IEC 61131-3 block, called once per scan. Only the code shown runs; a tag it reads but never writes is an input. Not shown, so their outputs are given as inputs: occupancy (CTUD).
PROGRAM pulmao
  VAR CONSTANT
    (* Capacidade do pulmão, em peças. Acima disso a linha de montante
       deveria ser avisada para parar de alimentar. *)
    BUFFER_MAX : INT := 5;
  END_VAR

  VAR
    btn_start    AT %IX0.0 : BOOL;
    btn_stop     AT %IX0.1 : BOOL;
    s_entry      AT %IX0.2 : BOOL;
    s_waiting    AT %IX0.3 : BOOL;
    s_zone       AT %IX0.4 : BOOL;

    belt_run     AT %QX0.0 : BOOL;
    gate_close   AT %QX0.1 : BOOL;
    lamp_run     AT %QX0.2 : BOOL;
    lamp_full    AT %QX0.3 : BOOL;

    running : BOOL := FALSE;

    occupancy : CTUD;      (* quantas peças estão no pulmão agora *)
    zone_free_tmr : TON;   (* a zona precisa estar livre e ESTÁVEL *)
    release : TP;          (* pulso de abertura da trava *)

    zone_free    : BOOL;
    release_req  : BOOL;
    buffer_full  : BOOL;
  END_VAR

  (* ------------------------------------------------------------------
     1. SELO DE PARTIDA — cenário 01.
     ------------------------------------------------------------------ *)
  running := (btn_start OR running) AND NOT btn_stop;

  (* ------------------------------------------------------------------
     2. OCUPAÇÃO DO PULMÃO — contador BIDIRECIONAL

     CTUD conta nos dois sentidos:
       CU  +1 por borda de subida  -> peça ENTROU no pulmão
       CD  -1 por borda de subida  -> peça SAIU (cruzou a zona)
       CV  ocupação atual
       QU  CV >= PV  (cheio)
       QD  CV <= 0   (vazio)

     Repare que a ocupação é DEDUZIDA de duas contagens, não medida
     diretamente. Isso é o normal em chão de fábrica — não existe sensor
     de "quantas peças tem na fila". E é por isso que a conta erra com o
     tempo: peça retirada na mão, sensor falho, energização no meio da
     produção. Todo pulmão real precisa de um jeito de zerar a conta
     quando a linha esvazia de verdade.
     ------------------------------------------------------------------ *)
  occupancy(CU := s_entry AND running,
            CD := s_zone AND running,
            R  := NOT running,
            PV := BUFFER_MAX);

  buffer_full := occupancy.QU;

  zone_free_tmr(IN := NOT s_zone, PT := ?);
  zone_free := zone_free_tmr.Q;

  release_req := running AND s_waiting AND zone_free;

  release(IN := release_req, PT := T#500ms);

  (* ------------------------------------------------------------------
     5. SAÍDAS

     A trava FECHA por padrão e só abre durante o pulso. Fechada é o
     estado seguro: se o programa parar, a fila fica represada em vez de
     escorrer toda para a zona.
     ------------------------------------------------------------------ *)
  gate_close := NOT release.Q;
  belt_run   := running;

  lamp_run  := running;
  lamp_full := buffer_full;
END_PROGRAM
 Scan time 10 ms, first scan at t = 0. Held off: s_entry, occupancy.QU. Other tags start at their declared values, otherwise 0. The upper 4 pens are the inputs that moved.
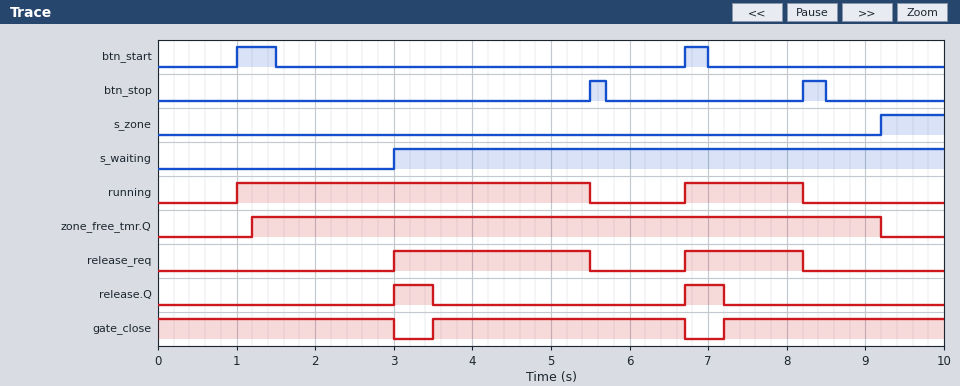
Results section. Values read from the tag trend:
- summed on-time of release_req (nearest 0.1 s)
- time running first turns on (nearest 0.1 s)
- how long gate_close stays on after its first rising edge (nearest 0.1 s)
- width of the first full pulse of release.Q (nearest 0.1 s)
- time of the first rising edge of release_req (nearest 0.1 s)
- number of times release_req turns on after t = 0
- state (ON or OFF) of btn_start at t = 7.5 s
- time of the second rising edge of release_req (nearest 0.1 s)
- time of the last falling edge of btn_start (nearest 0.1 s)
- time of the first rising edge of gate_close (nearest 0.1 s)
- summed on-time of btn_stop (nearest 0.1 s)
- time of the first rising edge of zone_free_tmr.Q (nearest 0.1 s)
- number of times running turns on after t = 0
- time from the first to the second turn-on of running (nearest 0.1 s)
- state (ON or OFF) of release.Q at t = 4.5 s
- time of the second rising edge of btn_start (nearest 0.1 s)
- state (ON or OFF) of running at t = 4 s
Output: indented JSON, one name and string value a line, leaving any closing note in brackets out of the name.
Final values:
{
  "summed on-time of release_req": "4.0 s",
  "time running first turns on": "1.0 s",
  "how long gate_close stays on after its first rising edge": "3.2 s",
  "width of the first full pulse of release.Q": "0.5 s",
  "time of the first rising edge of release_req": "3.0 s",
  "number of times release_req turns on after t = 0": "2",
  "state (ON or OFF) of btn_start at t = 7.5 s": "OFF",
  "time of the second rising edge of release_req": "6.7 s",
  "time of the last falling edge of btn_start": "7.0 s",
  "time of the first rising edge of gate_close": "3.5 s",
  "summed on-time of btn_stop": "0.5 s",
  "time of the first rising edge of zone_free_tmr.Q": "1.2 s",
  "number of times running turns on after t = 0": "2",
  "time from the first to the second turn-on of running": "5.7 s",
  "state (ON or OFF) of release.Q at t = 4.5 s": "OFF",
  "time of the second rising edge of btn_start": "6.7 s",
  "state (ON or OFF) of running at t = 4 s": "ON"
}
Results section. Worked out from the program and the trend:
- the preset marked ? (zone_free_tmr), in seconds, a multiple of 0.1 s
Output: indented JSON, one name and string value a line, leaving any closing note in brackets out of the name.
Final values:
{
  "the preset marked ? (zone_free_tmr), in seconds, a multiple of 0.1 s": "1.2 s"
}
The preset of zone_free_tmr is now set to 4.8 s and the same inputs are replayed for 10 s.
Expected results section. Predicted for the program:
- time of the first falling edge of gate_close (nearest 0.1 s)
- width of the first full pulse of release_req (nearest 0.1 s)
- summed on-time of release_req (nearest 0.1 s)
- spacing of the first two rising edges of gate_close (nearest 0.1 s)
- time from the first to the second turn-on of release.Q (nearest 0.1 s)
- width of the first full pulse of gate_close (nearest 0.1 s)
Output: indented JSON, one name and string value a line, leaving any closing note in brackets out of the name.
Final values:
{
  "time of the first falling edge of gate_close": "4.8 s",
  "width of the first full pulse of release_req": "0.7 s",
  "summed on-time of release_req": "2.2 s",
  "spacing of the first two rising edges of gate_close": "1.9 s",
  "time from the first to the second turn-on of release.Q": "1.9 s",
  "width of the first full pulse of gate_close": "1.4 s"
}
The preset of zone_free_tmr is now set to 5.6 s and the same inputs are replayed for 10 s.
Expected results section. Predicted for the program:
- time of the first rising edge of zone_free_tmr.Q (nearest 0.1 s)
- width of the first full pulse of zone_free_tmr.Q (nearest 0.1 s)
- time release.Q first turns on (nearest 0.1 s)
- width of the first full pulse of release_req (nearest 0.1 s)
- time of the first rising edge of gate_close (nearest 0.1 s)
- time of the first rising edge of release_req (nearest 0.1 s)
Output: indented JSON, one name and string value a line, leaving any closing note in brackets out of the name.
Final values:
{
  "time of the first rising edge of zone_free_tmr.Q": "5.6 s",
  "width of the first full pulse of zone_free_tmr.Q": "3.6 s",
  "time release.Q first turns on": "6.7 s",
  "width of the first full pulse of release_req": "1.5 s",
  "time of the first rising edge of gate_close": "7.2 s",
  "time of the first rising edge of release_req": "6.7 s"
}
